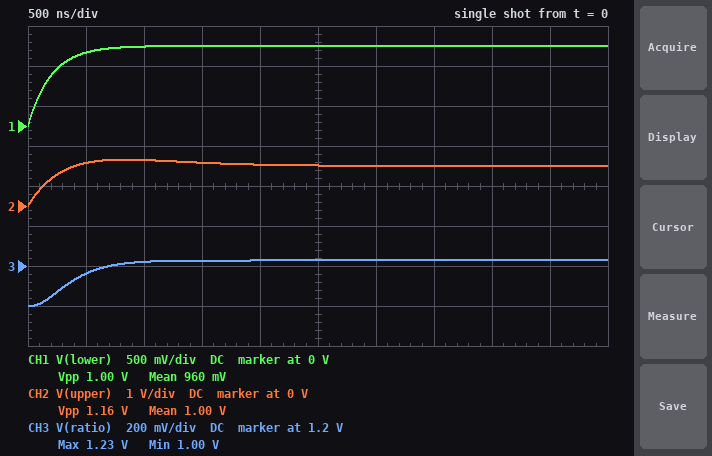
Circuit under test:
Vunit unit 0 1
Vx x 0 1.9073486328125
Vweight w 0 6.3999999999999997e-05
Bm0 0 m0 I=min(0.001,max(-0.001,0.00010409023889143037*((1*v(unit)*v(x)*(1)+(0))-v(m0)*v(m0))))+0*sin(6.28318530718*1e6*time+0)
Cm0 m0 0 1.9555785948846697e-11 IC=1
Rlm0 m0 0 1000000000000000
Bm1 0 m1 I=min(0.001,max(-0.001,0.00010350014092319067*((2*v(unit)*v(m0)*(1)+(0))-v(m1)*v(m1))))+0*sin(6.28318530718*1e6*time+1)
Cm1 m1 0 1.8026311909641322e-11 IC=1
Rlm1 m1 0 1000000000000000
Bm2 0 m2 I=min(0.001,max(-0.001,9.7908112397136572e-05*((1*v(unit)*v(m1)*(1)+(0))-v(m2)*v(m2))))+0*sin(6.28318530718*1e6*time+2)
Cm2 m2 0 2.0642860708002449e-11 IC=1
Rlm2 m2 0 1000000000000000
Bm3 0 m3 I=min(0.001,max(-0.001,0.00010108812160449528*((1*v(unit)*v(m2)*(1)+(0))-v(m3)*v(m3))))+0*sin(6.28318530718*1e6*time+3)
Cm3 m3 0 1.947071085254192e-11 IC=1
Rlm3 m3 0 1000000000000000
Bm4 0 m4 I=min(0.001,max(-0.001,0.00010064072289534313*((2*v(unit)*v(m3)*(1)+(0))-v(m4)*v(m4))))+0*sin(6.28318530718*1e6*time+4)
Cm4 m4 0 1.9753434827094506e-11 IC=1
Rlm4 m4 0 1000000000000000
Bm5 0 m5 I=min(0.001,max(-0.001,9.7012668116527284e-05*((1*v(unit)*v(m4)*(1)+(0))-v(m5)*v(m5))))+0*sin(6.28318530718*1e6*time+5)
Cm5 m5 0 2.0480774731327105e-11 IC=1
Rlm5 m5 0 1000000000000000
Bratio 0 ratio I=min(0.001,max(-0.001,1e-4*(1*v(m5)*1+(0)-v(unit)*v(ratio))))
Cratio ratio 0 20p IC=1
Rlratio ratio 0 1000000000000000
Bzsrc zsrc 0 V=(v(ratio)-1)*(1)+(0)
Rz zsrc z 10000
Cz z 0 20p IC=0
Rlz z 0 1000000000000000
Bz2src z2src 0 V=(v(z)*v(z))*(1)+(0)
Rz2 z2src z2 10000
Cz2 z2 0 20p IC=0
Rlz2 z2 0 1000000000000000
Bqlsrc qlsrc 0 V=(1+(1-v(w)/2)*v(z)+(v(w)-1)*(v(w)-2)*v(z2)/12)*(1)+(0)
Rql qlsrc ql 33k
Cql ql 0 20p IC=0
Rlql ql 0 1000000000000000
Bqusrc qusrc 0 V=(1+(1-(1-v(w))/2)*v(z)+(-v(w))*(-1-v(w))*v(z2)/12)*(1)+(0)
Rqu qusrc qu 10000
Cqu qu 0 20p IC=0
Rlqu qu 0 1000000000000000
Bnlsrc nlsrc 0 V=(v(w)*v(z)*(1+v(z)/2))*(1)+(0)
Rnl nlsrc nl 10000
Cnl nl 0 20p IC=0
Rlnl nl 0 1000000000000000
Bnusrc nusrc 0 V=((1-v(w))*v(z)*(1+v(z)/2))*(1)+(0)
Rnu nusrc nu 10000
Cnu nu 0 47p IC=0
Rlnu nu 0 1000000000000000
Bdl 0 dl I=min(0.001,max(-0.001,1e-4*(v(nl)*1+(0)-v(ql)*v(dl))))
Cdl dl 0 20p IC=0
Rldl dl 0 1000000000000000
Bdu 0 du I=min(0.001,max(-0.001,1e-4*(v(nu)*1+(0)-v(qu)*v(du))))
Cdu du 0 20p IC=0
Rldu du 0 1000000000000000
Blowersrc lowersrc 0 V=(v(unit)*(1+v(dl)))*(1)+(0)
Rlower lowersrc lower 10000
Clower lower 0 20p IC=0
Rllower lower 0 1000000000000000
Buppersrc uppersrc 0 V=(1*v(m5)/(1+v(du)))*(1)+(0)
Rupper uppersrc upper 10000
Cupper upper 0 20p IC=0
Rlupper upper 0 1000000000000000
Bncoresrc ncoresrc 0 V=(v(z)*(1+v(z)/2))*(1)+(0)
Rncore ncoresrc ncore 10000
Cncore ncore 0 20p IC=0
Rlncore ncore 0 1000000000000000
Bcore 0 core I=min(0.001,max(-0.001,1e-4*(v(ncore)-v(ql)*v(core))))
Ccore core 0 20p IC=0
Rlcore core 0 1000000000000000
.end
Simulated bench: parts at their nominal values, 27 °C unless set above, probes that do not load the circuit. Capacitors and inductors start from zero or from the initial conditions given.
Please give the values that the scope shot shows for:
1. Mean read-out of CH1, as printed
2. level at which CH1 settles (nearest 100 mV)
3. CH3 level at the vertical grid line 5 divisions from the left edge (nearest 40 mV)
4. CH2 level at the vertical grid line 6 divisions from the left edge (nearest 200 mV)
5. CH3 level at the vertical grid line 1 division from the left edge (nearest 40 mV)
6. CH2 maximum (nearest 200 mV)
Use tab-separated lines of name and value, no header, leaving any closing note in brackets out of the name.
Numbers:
Mean read-out of CH1, as printed	960 mV
level at which CH1 settles	1.0 V
CH3 level at the vertical grid line 5 divisions from the left edge	1.24 V
CH2 level at the vertical grid line 6 divisions from the left edge	1.0 V
CH3 level at the vertical grid line 1 division from the left edge	1.16 V
CH2 maximum	1.2 V
